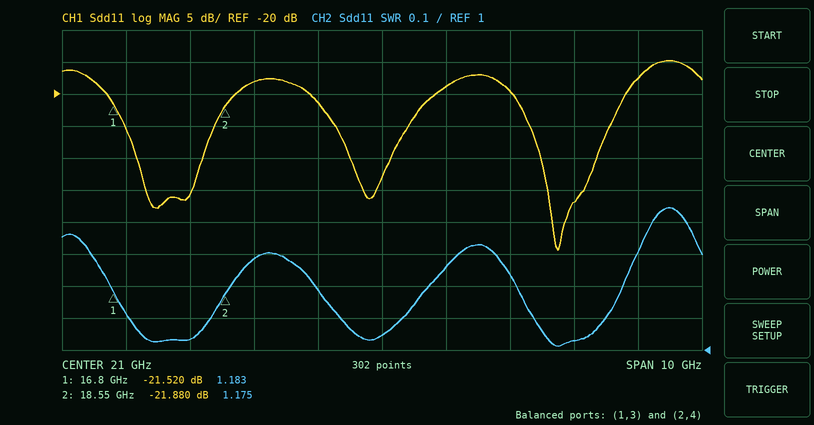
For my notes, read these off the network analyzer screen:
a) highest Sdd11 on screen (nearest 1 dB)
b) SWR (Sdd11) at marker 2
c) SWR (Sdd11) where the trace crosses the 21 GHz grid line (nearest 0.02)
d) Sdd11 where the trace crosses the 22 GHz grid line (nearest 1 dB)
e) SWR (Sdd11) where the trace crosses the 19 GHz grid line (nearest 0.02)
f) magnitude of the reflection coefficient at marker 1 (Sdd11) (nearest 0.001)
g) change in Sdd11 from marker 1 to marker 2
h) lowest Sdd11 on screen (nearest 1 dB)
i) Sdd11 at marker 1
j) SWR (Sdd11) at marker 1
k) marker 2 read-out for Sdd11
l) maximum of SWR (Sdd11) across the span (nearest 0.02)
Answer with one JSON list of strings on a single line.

["-15 dB", "1.175", "1.04", "-19 dB", "1.28", "0.084", "-0.360 dB", "-44 dB", "-21.520 dB", "1.183", "-21.880 dB", "1.44"]
